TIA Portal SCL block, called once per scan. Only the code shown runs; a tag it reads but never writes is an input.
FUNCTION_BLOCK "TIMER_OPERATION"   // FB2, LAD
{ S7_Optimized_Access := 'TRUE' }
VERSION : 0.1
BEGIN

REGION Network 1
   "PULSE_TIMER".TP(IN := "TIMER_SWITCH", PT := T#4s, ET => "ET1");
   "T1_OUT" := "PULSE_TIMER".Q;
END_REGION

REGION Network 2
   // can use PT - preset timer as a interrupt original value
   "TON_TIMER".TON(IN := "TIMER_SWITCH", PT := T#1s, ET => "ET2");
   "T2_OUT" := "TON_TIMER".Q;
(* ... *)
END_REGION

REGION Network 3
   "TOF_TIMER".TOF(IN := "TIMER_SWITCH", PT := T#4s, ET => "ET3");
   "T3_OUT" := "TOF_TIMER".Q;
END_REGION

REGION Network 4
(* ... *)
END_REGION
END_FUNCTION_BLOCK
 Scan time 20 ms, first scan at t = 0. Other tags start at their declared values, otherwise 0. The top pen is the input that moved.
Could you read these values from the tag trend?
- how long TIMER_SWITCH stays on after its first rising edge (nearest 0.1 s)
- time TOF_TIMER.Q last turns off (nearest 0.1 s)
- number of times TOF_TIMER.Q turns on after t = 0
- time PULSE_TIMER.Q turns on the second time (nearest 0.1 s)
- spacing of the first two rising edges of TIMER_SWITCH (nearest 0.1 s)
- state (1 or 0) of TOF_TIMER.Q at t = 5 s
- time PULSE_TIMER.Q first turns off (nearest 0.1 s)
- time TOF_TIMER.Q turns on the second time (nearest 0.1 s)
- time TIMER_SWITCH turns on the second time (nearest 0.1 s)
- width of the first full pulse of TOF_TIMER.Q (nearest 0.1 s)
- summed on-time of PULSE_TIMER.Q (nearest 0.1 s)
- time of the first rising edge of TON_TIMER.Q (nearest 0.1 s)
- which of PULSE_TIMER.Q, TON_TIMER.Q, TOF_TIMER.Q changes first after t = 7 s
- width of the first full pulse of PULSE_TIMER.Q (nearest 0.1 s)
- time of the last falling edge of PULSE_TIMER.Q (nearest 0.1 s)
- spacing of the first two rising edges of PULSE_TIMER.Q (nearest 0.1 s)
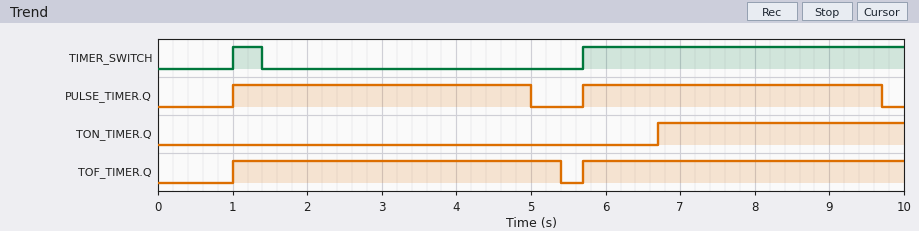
0.4 s
5.4 s
2
5.7 s
4.7 s
1
5.0 s
5.7 s
5.7 s
4.4 s
8.0 s
6.7 s
PULSE_TIMER.Q
4.0 s
9.7 s
4.7 s
